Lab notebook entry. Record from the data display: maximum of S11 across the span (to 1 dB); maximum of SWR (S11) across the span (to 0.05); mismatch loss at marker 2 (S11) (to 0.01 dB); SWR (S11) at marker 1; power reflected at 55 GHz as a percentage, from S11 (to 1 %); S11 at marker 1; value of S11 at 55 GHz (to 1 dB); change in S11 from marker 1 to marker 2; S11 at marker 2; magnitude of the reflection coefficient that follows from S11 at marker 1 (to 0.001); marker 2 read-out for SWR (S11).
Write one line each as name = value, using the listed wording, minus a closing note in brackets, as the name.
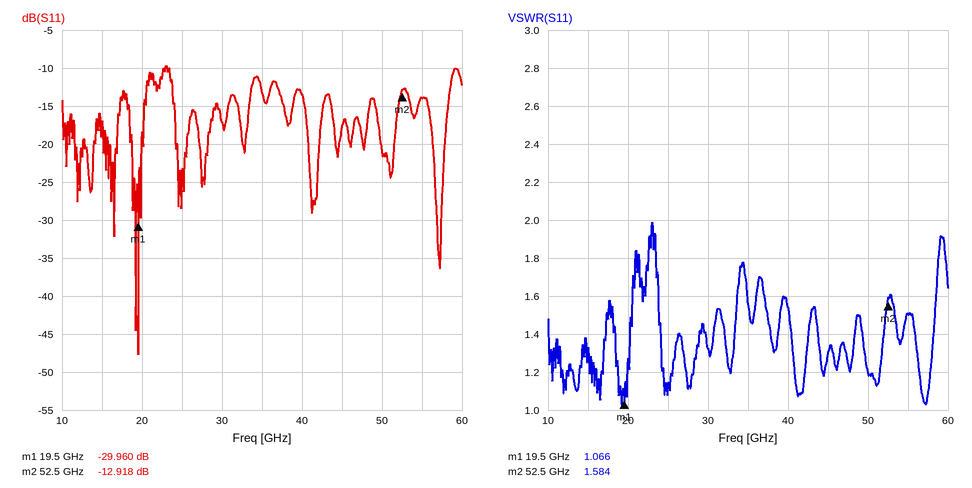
maximum of S11 across the span = -10 dB
maximum of SWR (S11) across the span = 2.00
mismatch loss at marker 2 (S11) = 0.23 dB
SWR (S11) at marker 1 = 1.066
power reflected at 55 GHz as a percentage, from S11 = 4 %
S11 at marker 1 = -29.960 dB
value of S11 at 55 GHz = -14 dB
change in S11 from marker 1 to marker 2 = 17.042 dB
S11 at marker 2 = -12.918 dB
magnitude of the reflection coefficient that follows from S11 at marker 1 = 0.032
marker 2 read-out for SWR = 1.584
